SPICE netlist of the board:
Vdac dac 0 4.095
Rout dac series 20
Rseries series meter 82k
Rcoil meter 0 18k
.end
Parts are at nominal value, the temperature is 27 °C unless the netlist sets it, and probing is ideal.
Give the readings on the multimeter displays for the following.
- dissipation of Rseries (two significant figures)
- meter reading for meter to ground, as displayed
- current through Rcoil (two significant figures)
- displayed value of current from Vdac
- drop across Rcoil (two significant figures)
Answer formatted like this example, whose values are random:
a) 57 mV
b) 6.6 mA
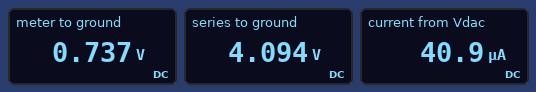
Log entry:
a) 140 µW
b) 0.737 V
c) 41 µA
d) 40.9 µA
e) 740 mV
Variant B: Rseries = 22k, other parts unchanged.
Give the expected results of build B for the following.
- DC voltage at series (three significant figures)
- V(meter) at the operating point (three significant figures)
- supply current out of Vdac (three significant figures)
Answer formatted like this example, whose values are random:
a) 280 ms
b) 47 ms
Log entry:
a) 4.09 V
b) 1.84 V
c) 102 µA
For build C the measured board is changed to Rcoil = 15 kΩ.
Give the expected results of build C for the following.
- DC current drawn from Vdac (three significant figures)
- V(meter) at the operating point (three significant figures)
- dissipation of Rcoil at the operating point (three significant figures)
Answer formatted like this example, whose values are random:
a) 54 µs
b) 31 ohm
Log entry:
a) 42.2 µA
b) 633 mV
c) 26.7 µW
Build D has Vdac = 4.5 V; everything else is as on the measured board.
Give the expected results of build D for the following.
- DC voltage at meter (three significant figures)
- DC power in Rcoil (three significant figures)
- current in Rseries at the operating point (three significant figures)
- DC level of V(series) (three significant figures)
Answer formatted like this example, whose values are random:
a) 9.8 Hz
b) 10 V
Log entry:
a) 810 mV
b) 36.4 µW
c) 45.0 µA
d) 4.50 V
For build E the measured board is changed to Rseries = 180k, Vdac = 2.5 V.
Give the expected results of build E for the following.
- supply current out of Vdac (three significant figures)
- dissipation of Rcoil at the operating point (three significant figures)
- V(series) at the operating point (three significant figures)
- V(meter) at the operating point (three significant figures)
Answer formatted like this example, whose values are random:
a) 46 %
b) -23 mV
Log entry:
a) 12.6 µA
b) 2.87 µW
c) 2.50 V
d) 227 mV
